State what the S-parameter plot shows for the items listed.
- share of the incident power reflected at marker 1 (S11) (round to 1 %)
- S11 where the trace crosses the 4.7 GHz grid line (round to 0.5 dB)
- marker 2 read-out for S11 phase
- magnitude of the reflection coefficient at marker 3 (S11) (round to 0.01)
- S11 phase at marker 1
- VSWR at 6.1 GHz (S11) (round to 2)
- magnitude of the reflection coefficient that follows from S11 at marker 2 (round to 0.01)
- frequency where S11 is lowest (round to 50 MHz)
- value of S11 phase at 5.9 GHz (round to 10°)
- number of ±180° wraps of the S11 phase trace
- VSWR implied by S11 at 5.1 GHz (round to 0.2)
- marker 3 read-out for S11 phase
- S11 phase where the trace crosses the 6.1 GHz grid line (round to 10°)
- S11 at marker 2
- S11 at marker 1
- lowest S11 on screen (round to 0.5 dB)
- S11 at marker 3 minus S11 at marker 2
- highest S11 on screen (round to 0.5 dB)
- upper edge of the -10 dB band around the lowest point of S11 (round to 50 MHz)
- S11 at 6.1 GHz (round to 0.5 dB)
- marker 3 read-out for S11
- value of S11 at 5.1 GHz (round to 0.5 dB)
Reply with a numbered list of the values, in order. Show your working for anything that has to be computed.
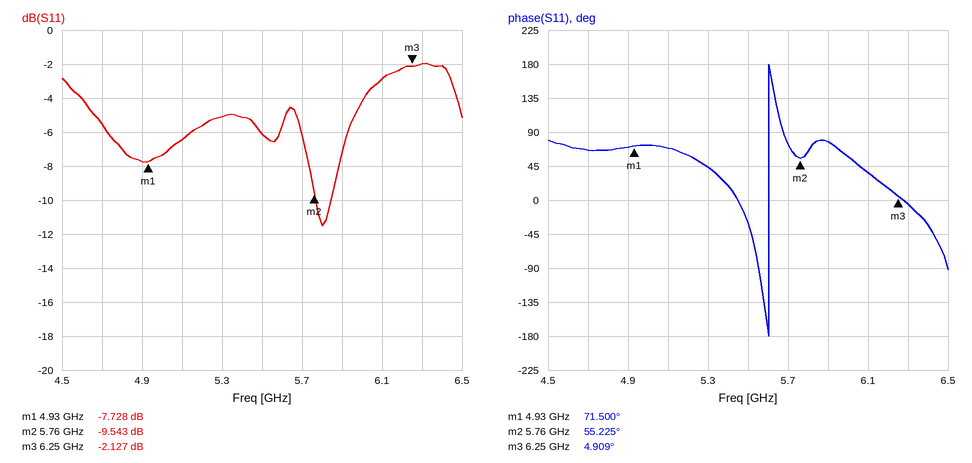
1. 10^(-7.728/10) ≈ 17 %
2. -5.5 dB
3. 55.225°
4. 10^(-2.127/20) ≈ 0.78
5. 71.500°
6. |Γ| = 10^(-3/20) = 0.7079; VSWR = (1 + 0.7079)/(1 − 0.7079) ≈ 6
7. 10^(-9.543/20) ≈ 0.33
8. 5.80 GHz
9. 80°
10. 1
11. |Γ| = 10^(-6.5/20) = 0.4732; VSWR = (1 + 0.4732)/(1 − 0.4732) ≈ 2.8
12. 4.909°
13. 40°
14. -9.543 dB
15. -7.728 dB
16. -11.5 dB
17. -2.127 − (-9.543) = 7.416 dB
18. -2.0 dB
19. 5.85 GHz
20. -3.0 dB
21. -2.127 dB
22. -6.5 dB
